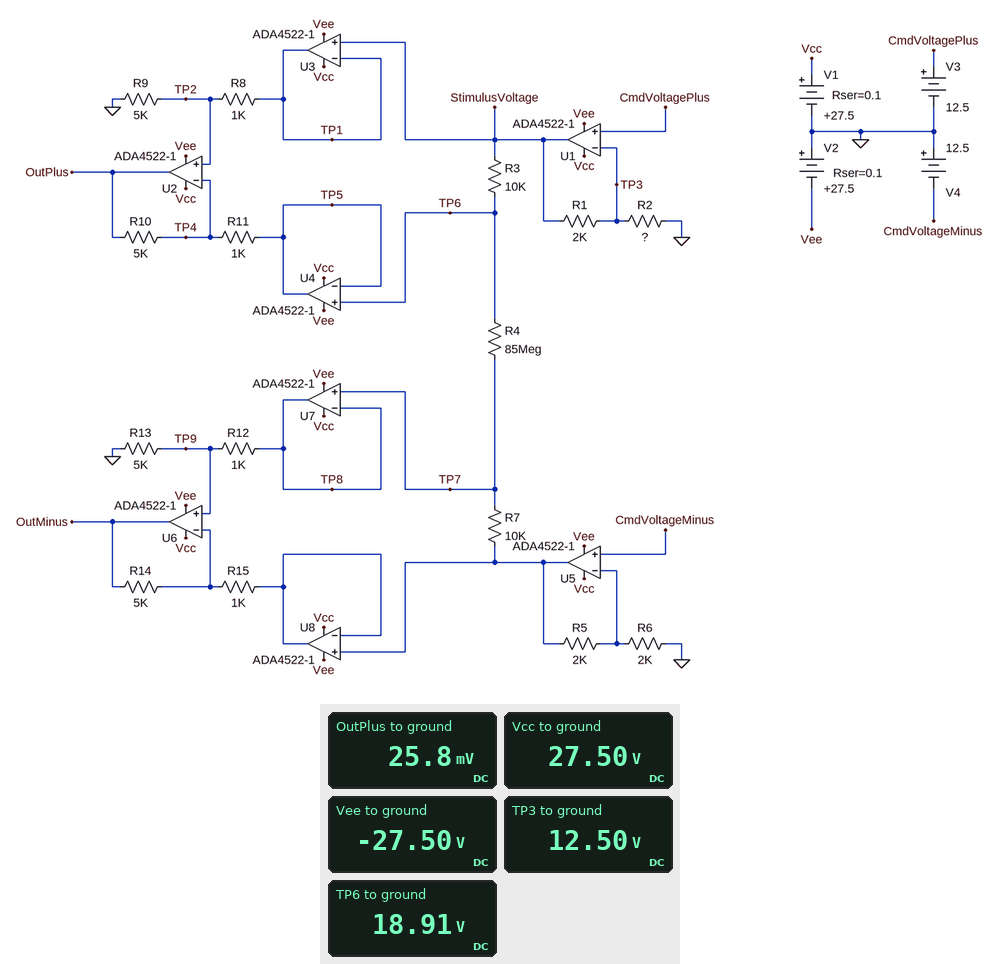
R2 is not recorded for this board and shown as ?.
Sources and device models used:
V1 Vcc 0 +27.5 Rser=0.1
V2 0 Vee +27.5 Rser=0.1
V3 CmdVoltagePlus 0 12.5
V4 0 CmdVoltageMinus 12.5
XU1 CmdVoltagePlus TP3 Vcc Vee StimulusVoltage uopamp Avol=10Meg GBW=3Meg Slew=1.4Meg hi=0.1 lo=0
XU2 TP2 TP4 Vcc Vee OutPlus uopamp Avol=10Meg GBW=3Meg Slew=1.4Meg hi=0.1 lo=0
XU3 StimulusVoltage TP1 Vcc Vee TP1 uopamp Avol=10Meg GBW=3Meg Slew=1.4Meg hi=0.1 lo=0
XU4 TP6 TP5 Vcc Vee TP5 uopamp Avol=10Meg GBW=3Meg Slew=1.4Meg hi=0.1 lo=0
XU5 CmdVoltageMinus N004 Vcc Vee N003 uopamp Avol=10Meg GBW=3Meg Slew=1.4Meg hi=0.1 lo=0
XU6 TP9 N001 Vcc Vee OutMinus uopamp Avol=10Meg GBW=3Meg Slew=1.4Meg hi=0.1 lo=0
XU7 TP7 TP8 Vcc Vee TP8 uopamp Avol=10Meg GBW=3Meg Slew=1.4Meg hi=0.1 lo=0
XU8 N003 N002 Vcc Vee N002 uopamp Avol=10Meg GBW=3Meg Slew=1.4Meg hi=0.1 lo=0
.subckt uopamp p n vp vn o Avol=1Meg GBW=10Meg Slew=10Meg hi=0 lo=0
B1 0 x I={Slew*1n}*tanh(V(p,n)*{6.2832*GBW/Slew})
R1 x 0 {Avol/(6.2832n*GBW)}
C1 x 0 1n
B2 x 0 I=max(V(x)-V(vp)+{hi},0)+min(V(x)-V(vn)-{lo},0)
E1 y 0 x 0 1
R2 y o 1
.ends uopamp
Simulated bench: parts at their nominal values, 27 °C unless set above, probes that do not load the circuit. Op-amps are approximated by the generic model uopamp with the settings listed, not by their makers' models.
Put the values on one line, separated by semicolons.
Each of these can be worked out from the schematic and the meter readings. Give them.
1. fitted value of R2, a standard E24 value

3.9 kΩ
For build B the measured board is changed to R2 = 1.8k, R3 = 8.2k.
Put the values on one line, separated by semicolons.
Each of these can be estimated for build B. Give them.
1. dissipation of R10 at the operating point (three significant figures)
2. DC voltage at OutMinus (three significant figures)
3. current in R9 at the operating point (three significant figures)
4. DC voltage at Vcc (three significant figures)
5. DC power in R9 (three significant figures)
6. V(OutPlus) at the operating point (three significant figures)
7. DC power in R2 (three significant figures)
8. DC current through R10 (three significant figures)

96.5 mW; 30.2 mV; 4.40 mA; 27.5 V; 96.7 mW; 24.8 mV; 86.8 mW; 4.39 mA
